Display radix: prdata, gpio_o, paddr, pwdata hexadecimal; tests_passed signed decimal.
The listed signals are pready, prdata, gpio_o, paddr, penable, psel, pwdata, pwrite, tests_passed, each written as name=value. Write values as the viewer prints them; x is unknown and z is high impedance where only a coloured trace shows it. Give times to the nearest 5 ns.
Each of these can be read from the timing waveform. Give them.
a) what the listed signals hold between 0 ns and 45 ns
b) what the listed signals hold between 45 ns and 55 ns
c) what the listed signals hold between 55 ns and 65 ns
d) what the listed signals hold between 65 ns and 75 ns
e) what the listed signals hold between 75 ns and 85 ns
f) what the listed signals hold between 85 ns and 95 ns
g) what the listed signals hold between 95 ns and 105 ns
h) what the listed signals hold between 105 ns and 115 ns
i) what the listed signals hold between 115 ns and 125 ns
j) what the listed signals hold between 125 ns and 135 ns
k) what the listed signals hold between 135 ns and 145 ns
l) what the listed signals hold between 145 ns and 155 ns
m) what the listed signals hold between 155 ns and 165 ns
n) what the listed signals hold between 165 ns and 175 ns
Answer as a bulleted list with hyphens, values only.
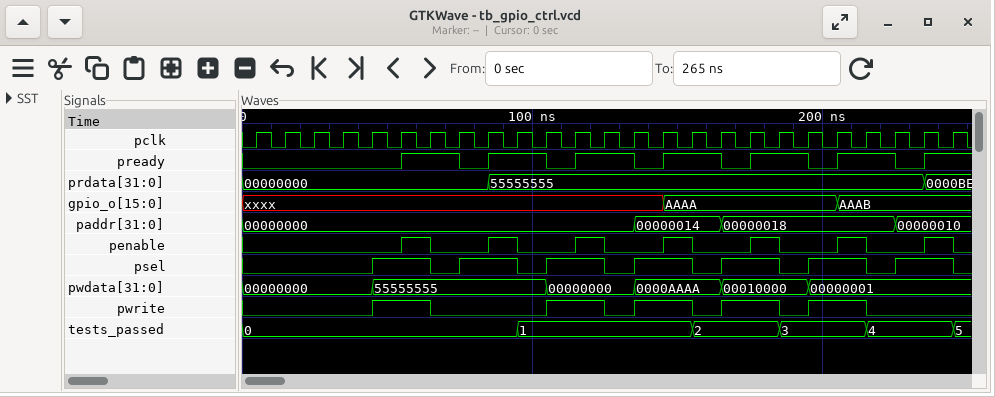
- pready=0, prdata=00000000, gpio_o=xxxx, paddr=00000000, penable=0, psel=0, pwdata=00000000, pwrite=0, tests_passed=0
- pready=0, prdata=00000000, gpio_o=xxxx, paddr=00000000, penable=0, psel=1, pwdata=55555555, pwrite=1, tests_passed=0
- pready=1, prdata=00000000, gpio_o=xxxx, paddr=00000000, penable=1, psel=1, pwdata=55555555, pwrite=1, tests_passed=0
- pready=1, prdata=00000000, gpio_o=xxxx, paddr=00000000, penable=0, psel=0, pwdata=55555555, pwrite=0, tests_passed=0
- pready=0, prdata=00000000, gpio_o=xxxx, paddr=00000000, penable=0, psel=1, pwdata=55555555, pwrite=0, tests_passed=0
- pready=1, prdata=55555555, gpio_o=xxxx, paddr=00000000, penable=1, psel=1, pwdata=55555555, pwrite=0, tests_passed=0
- pready=1, prdata=55555555, gpio_o=xxxx, paddr=00000000, penable=0, psel=0, pwdata=55555555, pwrite=0, tests_passed=1
- pready=0, prdata=55555555, gpio_o=xxxx, paddr=00000000, penable=0, psel=1, pwdata=00000000, pwrite=1, tests_passed=1
- pready=1, prdata=55555555, gpio_o=xxxx, paddr=00000000, penable=1, psel=1, pwdata=00000000, pwrite=1, tests_passed=1
- pready=1, prdata=55555555, gpio_o=xxxx, paddr=00000000, penable=0, psel=0, pwdata=00000000, pwrite=0, tests_passed=1
- pready=0, prdata=55555555, gpio_o=xxxx, paddr=00000014, penable=0, psel=1, pwdata=0000AAAA, pwrite=1, tests_passed=1
- pready=1, prdata=55555555, gpio_o=AAAA, paddr=00000014, penable=1, psel=1, pwdata=0000AAAA, pwrite=1, tests_passed=1
- pready=1, prdata=55555555, gpio_o=AAAA, paddr=00000014, penable=0, psel=0, pwdata=0000AAAA, pwrite=0, tests_passed=2
- pready=0, prdata=55555555, gpio_o=AAAA, paddr=00000018, penable=0, psel=1, pwdata=00010000, pwrite=1, tests_passed=2
